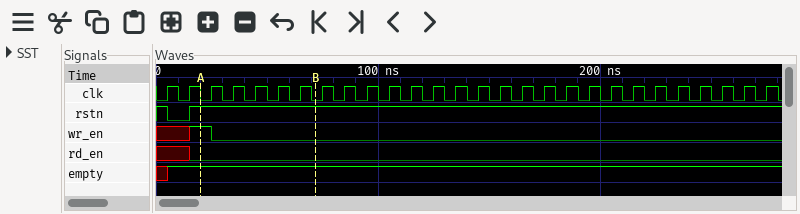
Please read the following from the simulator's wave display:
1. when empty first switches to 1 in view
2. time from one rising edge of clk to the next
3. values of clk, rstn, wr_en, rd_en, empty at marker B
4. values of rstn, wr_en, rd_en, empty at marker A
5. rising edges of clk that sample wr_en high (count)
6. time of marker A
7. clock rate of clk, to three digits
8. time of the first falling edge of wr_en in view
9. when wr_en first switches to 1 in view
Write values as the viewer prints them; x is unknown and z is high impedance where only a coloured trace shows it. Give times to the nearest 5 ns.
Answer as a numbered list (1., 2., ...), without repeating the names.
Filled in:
1. 5 ns
2. 10 ns
3. clk=0, rstn=1, wr_en=0, rd_en=0, empty=1
4. rstn=1, wr_en=1, rd_en=0, empty=1
5. 1
6. 20 ns
7. 100 MHz
8. 25 ns
9. 15 ns
